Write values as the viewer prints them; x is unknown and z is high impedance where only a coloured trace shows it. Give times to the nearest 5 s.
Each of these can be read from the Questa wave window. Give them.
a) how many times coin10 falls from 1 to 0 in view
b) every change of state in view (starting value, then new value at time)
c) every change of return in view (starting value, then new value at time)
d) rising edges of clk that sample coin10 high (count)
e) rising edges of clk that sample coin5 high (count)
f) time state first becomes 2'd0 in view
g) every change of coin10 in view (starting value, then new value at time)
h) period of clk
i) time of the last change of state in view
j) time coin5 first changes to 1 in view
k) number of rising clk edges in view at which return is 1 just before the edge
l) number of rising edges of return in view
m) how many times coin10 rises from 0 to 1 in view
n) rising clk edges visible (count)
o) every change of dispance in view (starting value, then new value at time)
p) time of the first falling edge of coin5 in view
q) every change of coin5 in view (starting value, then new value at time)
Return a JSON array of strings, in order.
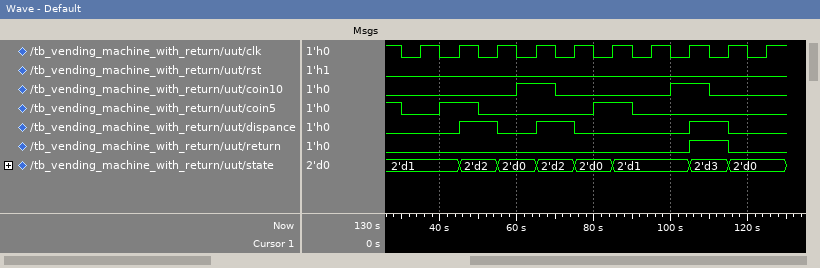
["2", "2'd1, 2'd2 at 45 s, 2'd0 at 55 s, 2'd2 at 65 s, 2'd0 at 75 s, 2'd1 at 85 s, 2'd3 at 105 s, 2'd0 at 115 s", "0, 1 at 105 s, 0 at 115 s", "2", "2", "55 s", "0, 1 at 60 s, 0 at 70 s, 1 at 100 s, 0 at 110 s", "10 s", "115 s", "40 s", "1", "1", "2", "10", "0, 1 at 45 s, 0 at 55 s, 1 at 65 s, 0 at 75 s, 1 at 105 s, 0 at 115 s", "30 s", "1, 0 at 30 s, 1 at 40 s, 0 at 50 s, 1 at 80 s, 0 at 90 s"]
